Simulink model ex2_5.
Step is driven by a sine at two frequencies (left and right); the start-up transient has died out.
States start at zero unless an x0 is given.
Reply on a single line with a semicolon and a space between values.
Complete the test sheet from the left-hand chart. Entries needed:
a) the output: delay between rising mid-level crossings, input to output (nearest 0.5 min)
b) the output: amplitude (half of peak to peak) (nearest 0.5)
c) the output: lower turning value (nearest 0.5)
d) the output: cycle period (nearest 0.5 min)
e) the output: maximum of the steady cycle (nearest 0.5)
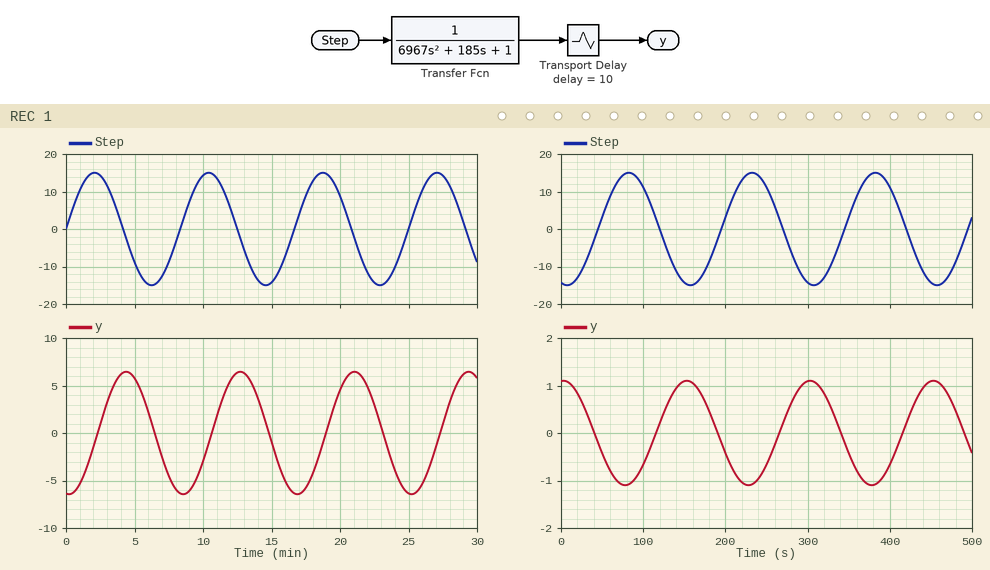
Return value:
2.5 min; 6.5; -6.5; 8.5 min; 6.5
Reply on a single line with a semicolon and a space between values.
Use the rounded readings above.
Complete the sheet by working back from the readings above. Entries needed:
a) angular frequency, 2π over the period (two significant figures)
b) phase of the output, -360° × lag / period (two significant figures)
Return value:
0.74 rad/min; -110°
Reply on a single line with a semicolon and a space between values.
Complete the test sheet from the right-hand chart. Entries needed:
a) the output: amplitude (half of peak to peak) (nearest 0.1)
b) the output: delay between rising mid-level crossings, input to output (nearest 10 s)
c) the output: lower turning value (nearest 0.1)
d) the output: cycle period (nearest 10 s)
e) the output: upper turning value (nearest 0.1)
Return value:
1.1; 70 s; -1.1; 150 s; 1.1
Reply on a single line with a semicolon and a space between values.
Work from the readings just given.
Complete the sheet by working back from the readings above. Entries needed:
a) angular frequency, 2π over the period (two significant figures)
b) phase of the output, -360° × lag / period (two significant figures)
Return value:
0.042 rad/s; -170°
